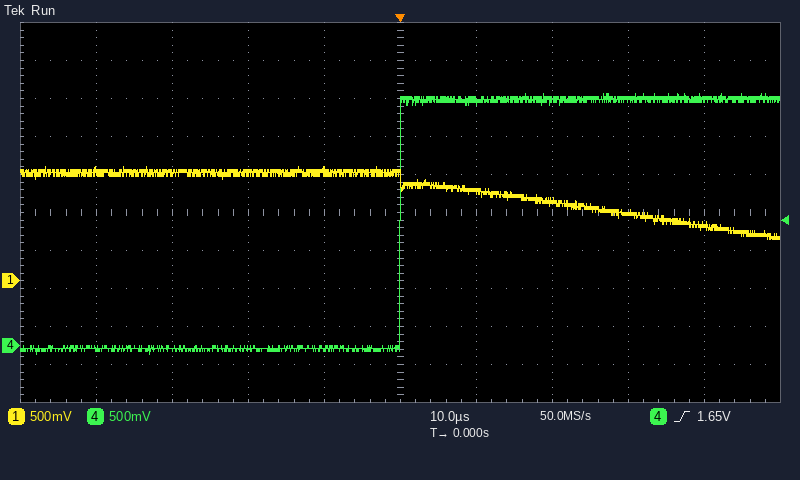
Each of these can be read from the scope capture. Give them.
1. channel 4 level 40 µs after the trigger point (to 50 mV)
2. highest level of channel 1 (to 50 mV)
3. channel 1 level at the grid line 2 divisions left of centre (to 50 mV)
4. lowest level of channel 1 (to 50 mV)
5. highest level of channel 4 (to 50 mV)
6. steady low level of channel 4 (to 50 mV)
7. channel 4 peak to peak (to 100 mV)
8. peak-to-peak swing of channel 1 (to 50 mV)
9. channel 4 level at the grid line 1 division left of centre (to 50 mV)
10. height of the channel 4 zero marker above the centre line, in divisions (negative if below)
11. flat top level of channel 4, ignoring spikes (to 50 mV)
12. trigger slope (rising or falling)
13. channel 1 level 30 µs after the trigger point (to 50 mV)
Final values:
3.25 V
1.50 V
1.40 V
550 mV
3.30 V
-50 mV
3.40 V
950 mV
-50 mV
-3.5 div
3.25 V
rising
900 mV
